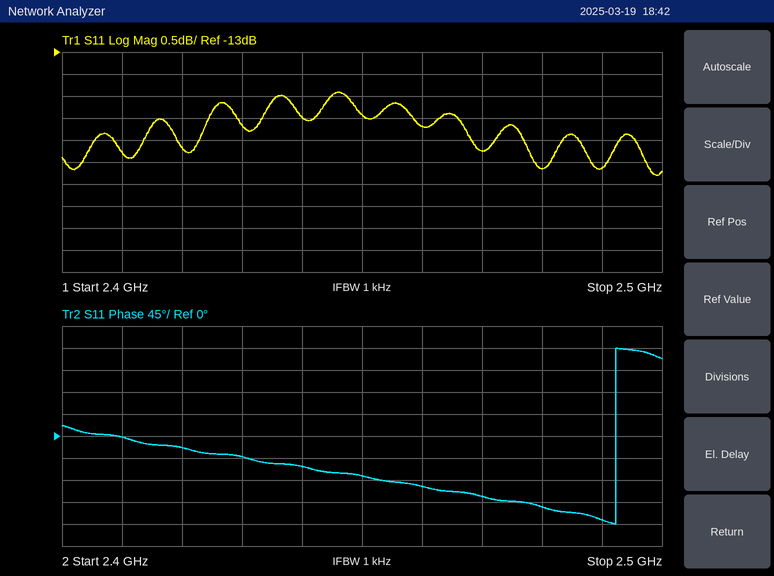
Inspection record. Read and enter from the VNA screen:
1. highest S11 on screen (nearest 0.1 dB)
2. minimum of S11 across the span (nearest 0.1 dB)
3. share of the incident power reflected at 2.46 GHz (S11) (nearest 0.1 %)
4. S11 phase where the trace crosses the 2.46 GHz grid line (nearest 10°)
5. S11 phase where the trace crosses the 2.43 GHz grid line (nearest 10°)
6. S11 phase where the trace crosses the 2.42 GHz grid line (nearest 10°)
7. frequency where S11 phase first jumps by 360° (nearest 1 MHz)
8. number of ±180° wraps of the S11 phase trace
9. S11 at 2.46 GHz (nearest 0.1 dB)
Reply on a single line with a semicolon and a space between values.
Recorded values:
-13.9 dB; -15.8 dB; 3.4 %; -100°; -40°; -20°; 2.492 GHz; 1; -14.7 dB
